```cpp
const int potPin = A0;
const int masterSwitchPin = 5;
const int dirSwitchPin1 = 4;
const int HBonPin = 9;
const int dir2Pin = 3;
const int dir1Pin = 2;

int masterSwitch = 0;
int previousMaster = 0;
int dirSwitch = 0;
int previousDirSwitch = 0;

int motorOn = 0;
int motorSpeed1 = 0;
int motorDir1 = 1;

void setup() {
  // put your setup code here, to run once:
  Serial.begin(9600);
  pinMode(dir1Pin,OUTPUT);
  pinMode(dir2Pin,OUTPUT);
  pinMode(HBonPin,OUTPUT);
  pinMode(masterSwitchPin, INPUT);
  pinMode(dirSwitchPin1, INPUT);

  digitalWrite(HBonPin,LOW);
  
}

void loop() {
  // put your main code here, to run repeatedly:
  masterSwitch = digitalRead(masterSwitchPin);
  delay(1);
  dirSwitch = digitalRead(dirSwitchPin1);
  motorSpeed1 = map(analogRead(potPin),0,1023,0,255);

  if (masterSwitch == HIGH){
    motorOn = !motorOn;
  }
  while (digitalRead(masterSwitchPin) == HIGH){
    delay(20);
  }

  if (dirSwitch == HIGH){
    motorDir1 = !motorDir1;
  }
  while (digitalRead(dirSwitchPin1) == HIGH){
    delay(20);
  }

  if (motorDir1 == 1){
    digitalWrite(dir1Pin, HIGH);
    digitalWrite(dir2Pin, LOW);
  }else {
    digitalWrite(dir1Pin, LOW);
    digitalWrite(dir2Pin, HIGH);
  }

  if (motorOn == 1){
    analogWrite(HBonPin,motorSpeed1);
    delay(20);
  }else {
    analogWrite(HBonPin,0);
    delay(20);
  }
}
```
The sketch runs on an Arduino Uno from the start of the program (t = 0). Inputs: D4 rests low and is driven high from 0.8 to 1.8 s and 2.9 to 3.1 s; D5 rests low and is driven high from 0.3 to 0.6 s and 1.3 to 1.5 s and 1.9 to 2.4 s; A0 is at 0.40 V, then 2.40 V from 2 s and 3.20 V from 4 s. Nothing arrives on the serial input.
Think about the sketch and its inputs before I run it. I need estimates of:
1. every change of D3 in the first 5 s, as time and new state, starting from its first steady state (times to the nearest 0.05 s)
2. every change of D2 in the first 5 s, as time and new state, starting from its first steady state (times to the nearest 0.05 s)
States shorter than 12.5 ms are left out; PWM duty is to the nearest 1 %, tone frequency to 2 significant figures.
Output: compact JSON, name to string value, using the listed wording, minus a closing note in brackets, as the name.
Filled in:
{"every change of D3 in the first 5 s, as time and new state, starting from its first steady state": "0 s low; 1.8 s high; 3.1 s low", "every change of D2 in the first 5 s, as time and new state, starting from its first steady state": "0 s high; 1.8 s low; 3.1 s high"}
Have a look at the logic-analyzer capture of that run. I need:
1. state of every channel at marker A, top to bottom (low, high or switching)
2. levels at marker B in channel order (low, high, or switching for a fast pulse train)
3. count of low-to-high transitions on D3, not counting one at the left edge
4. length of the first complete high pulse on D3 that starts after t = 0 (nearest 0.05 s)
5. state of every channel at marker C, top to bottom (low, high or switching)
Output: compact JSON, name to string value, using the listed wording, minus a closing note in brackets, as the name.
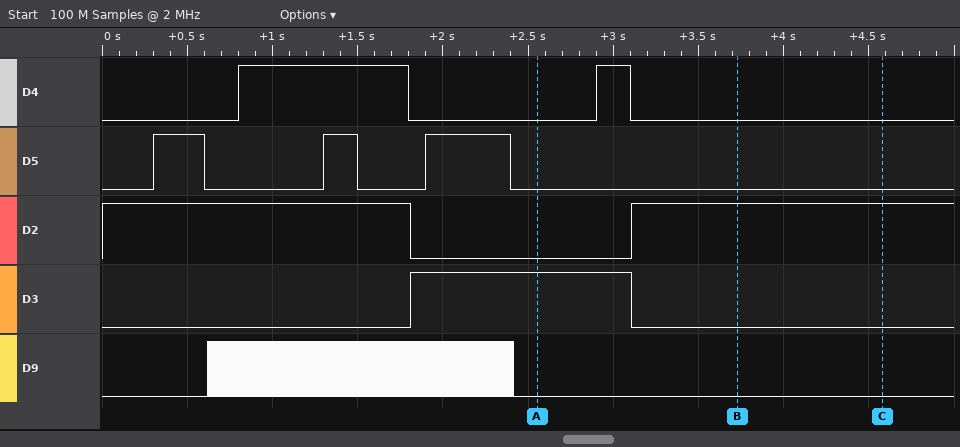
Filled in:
{"state of every channel at marker A, top to bottom": "D4 low, D5 low, D2 low, D3 high, D9 low", "levels at marker B in channel order": "D4 low, D5 low, D2 high, D3 low, D9 low", "count of low-to-high transitions on D3, not counting one at the left edge": "1", "length of the first complete high pulse on D3 that starts after t = 0": "1.30 s", "state of every channel at marker C, top to bottom": "D4 low, D5 low, D2 high, D3 low, D9 low"}
